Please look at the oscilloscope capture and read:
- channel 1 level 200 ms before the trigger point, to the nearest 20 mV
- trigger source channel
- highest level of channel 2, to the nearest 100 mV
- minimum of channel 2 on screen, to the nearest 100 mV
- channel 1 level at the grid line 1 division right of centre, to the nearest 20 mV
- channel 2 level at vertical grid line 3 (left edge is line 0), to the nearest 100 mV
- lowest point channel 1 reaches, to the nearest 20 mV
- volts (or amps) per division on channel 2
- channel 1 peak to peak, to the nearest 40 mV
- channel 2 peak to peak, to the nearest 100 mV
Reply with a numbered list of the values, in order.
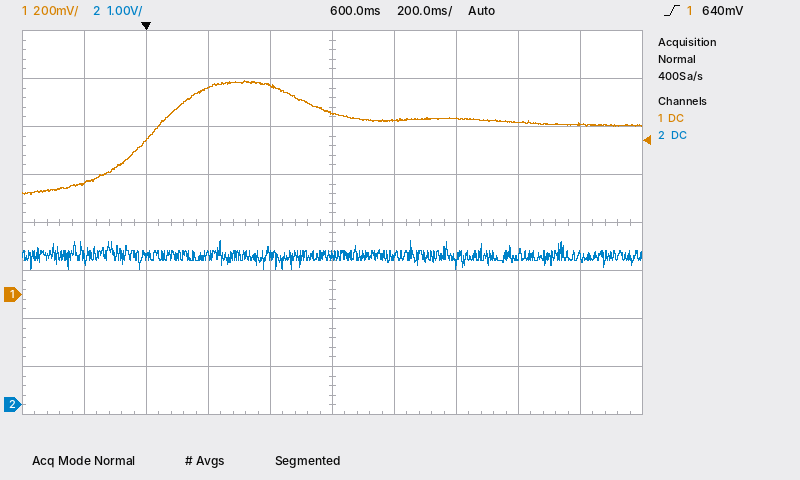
1. 460 mV
2. channel 1
3. 3.4 V
4. 2.8 V
5. 720 mV
6. 3.1 V
7. 420 mV
8. 1 V
9. 480 mV
10. 600 mV
